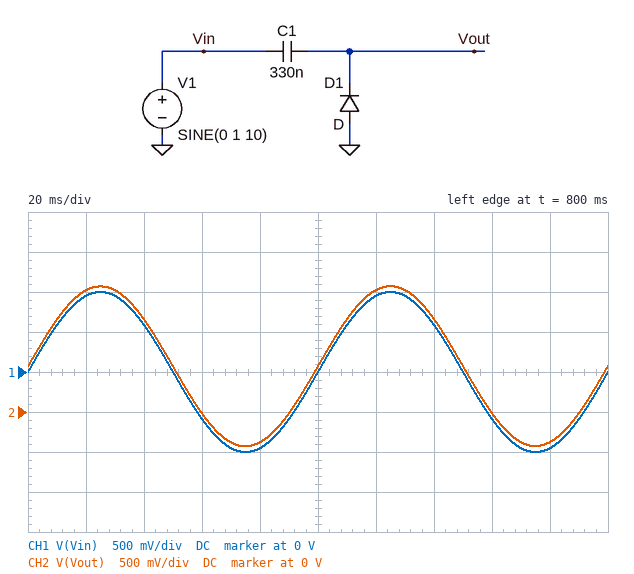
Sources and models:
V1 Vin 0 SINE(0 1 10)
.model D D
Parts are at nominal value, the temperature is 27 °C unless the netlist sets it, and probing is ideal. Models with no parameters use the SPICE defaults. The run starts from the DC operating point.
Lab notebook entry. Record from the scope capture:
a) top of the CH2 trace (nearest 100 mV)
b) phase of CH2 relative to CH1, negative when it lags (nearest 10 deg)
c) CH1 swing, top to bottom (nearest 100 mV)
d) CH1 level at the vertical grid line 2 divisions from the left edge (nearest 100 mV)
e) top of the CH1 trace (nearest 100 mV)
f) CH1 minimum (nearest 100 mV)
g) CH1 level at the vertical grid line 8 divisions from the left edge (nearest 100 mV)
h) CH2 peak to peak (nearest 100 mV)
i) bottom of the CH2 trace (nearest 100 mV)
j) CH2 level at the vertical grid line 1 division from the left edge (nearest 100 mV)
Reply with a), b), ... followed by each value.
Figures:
a) 1.6 V
b) 0 deg
c) 2.0 V
d) 600 mV
e) 1.0 V
f) -1.0 V
g) -600 mV
h) 2.0 V
i) -400 mV
j) 1.5 V
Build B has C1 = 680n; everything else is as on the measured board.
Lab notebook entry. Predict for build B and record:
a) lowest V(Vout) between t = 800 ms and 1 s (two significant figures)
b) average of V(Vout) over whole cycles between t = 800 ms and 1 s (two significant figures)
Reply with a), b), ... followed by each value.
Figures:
a) -450 mV
b) 550 mV
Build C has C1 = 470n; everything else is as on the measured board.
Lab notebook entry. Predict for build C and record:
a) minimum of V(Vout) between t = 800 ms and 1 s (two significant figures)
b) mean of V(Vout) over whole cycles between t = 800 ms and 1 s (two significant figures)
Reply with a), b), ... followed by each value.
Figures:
a) -440 mV
b) 560 mV
